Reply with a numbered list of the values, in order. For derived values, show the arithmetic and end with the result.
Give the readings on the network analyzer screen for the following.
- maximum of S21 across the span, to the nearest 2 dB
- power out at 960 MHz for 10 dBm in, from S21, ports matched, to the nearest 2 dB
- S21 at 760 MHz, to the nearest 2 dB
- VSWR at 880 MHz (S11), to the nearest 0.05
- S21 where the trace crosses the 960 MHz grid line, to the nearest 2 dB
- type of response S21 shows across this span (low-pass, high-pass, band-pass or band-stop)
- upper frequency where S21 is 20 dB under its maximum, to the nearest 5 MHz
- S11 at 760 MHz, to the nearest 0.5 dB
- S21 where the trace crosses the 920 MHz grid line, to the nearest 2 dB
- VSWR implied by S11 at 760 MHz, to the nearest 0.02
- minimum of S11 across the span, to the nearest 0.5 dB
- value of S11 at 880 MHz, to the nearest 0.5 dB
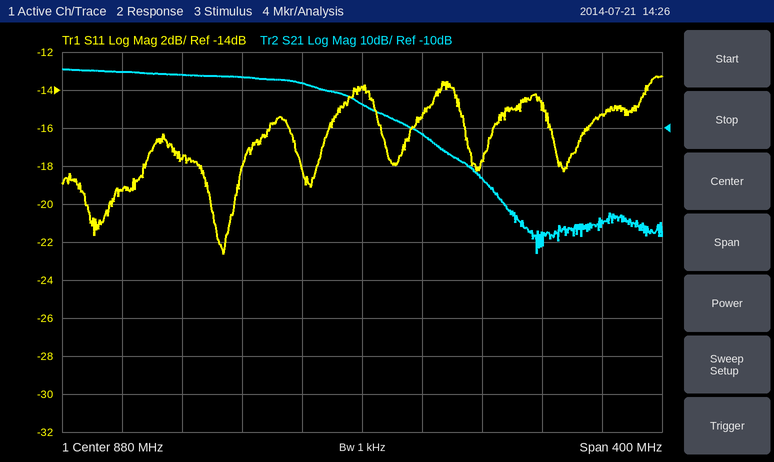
1. 6 dB
2. 10 dBm + (-24 dB) = -14 dBm
3. 4 dB
4. |Γ| = 10^(-14/20) = 0.1995; VSWR = (1 + 0.1995)/(1 − 0.1995) ≈ 1.50
5. -24 dB
6. low-pass
7. 930 MHz
8. -17.5 dB
9. -12 dB
10. |Γ| = 10^(-17.5/20) = 0.1334; VSWR = (1 + 0.1334)/(1 − 0.1334) ≈ 1.31, so 1.30 to the nearest 0.02
11. -22.5 dB
12. -14.0 dB
